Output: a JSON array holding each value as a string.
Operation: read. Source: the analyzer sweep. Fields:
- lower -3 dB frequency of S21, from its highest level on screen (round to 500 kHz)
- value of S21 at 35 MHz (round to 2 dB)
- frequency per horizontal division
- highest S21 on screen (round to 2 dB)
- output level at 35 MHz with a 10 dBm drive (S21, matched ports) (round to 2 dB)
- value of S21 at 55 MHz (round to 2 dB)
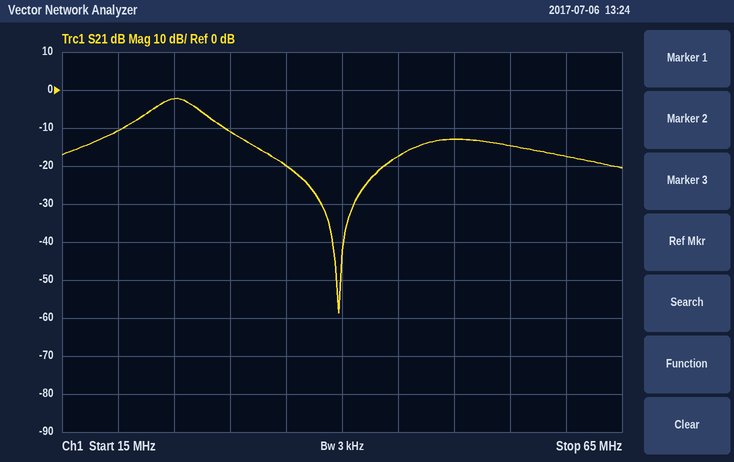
["23.0 MHz", "-20 dB", "5 MHz", "-2 dB", "-10 dBm", "-14 dB"]
